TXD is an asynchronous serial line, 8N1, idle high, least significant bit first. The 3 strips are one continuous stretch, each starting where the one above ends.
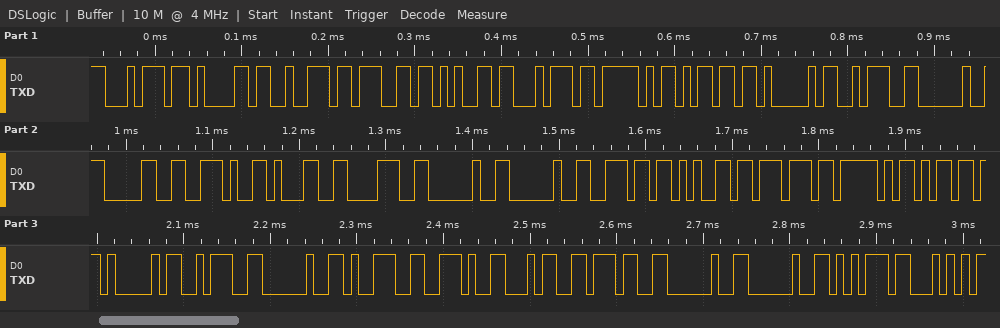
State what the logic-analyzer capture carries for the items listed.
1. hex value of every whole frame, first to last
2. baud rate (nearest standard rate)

74 61 72 67 65 74 5F 6D 41 3A 20 30 2E 31 38 20 20 6E 65 77 5F 6D 41 3A 20 39 2E 34 37 20 20 75 54
115200 baud
